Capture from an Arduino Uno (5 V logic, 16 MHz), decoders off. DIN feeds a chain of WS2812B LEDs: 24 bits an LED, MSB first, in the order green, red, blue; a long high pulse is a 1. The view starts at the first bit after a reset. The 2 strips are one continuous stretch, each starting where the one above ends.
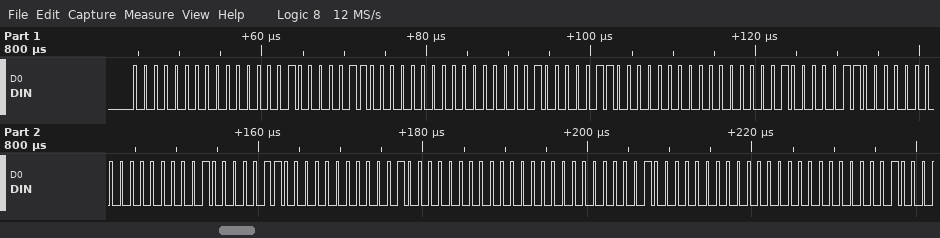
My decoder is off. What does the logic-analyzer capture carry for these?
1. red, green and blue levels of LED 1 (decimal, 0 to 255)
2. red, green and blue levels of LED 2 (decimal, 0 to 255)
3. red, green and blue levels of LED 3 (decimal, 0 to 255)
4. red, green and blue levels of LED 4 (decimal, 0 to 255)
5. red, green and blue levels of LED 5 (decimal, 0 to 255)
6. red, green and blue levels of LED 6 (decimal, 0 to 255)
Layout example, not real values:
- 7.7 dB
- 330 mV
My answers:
- 1, 0, 6
- 1, 0, 6
- 1, 0, 6
- 1, 0, 6
- 32, 0, 0
- 32, 0, 0
